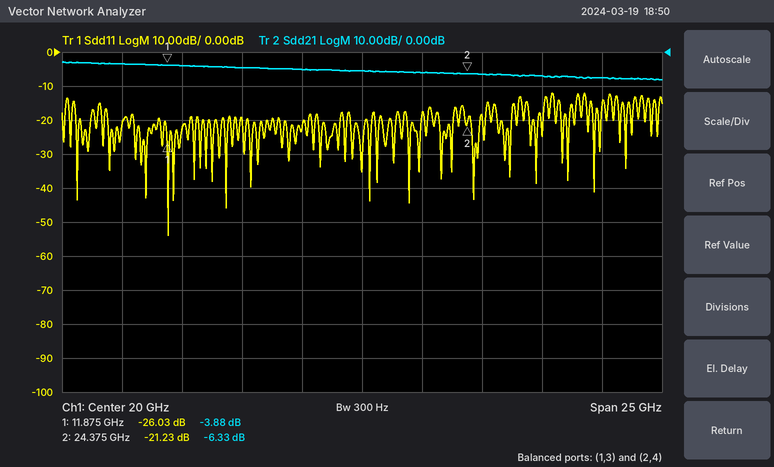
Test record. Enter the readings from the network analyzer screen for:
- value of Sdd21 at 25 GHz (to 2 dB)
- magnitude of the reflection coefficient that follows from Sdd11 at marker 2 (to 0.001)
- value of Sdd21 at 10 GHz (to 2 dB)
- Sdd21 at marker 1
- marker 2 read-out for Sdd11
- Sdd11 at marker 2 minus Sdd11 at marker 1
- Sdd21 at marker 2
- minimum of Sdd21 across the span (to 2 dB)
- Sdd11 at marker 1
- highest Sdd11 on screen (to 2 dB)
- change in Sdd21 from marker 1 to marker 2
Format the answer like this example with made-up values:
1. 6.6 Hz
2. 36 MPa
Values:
1. -6 dB
2. 0.087
3. -4 dB
4. -3.88 dB
5. -21.23 dB
6. 4.80 dB
7. -6.33 dB
8. -8 dB
9. -26.03 dB
10. -12 dB
11. -2.45 dB
